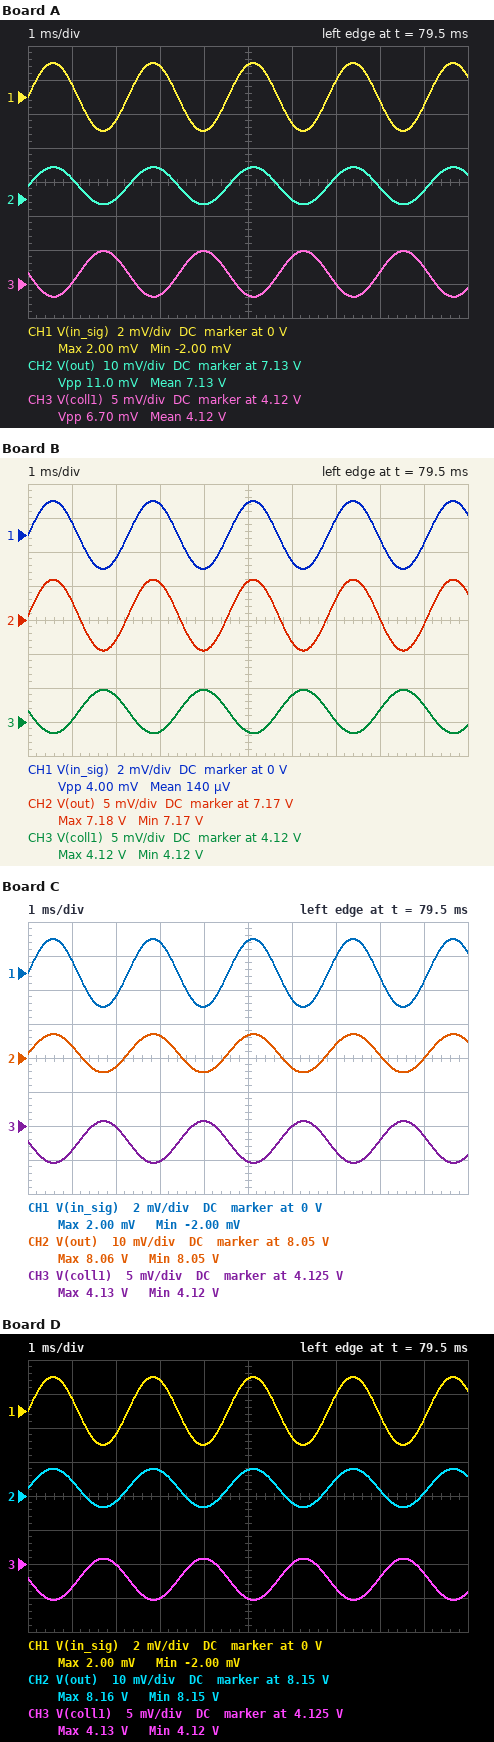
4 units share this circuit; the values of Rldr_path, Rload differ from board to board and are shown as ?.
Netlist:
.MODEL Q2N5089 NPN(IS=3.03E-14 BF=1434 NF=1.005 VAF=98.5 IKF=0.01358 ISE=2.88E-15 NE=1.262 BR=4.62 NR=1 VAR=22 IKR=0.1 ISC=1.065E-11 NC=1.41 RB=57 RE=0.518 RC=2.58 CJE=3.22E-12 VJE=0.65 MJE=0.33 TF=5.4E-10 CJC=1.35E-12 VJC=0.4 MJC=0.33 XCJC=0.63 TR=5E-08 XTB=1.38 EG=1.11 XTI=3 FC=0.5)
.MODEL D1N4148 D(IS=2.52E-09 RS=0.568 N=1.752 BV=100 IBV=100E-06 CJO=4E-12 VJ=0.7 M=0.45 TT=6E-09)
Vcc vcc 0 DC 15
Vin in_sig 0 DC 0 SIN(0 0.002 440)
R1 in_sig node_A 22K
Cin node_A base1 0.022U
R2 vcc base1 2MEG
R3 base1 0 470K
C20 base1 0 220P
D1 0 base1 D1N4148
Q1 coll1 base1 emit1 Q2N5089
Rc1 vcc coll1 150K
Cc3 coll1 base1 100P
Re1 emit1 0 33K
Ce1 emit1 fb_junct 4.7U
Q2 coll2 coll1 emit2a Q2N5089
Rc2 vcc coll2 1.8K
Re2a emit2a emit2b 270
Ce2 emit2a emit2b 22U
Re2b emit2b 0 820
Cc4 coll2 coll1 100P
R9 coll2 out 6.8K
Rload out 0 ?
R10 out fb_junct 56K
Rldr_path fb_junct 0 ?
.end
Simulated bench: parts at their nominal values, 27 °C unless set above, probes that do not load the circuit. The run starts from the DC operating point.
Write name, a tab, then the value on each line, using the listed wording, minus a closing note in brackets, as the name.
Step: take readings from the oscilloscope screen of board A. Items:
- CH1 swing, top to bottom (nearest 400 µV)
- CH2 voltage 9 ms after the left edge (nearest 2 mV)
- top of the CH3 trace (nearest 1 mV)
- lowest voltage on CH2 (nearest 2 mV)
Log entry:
CH1 swing, top to bottom	4.0 mV
CH2 voltage 9 ms after the left edge	7.132 V
top of the CH3 trace	4.125 V
lowest voltage on CH2	7.128 V
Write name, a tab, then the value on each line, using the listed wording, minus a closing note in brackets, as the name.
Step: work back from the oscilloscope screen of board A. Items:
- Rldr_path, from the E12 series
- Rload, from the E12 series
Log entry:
Rldr_path, from the E12 series	47 kΩ
Rload, from the E12 series	39 kΩ
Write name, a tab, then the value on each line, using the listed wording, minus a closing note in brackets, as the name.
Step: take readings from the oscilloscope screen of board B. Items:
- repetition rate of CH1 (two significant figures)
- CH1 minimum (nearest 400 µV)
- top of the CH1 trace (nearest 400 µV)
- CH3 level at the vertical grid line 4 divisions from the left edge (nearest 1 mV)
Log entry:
repetition rate of CH1	440 Hz
CH1 minimum	-2.0 mV
top of the CH1 trace	2.0 mV
CH3 level at the vertical grid line 4 divisions from the left edge	4.125 V
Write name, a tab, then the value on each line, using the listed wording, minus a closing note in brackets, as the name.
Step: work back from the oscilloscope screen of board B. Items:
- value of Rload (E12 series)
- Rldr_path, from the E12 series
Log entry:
value of Rload	39 kΩ
Rldr_path, from the E12 series	56 kΩ
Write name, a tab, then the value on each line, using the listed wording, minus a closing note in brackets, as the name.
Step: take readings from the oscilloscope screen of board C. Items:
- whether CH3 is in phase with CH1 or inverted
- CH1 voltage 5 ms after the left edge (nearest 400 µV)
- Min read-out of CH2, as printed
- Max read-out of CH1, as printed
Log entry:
whether CH3 is in phase with CH1 or inverted	inverted
CH1 voltage 5 ms after the left edge	2.0 mV
Min read-out of CH2, as printed	8.05 V
Max read-out of CH1, as printed	2.00 mV
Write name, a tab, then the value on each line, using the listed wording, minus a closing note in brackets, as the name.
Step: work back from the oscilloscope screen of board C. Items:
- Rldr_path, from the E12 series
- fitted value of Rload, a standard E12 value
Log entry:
Rldr_path, from the E12 series	47 kΩ
fitted value of Rload, a standard E12 value	120 kΩ
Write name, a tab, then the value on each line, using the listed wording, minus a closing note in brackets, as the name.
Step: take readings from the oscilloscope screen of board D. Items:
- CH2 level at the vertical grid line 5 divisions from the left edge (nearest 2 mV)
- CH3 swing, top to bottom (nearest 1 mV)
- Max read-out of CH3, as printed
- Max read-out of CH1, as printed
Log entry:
CH2 level at the vertical grid line 5 divisions from the left edge	8.158 V
CH3 swing, top to bottom	6 mV
Max read-out of CH3, as printed	4.13 V
Max read-out of CH1, as printed	2.00 mV
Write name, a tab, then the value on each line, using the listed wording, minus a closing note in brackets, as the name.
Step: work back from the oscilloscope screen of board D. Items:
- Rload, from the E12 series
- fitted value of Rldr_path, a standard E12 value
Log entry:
Rload, from the E12 series	150 kΩ
fitted value of Rldr_path, a standard E12 value	47 kΩ
